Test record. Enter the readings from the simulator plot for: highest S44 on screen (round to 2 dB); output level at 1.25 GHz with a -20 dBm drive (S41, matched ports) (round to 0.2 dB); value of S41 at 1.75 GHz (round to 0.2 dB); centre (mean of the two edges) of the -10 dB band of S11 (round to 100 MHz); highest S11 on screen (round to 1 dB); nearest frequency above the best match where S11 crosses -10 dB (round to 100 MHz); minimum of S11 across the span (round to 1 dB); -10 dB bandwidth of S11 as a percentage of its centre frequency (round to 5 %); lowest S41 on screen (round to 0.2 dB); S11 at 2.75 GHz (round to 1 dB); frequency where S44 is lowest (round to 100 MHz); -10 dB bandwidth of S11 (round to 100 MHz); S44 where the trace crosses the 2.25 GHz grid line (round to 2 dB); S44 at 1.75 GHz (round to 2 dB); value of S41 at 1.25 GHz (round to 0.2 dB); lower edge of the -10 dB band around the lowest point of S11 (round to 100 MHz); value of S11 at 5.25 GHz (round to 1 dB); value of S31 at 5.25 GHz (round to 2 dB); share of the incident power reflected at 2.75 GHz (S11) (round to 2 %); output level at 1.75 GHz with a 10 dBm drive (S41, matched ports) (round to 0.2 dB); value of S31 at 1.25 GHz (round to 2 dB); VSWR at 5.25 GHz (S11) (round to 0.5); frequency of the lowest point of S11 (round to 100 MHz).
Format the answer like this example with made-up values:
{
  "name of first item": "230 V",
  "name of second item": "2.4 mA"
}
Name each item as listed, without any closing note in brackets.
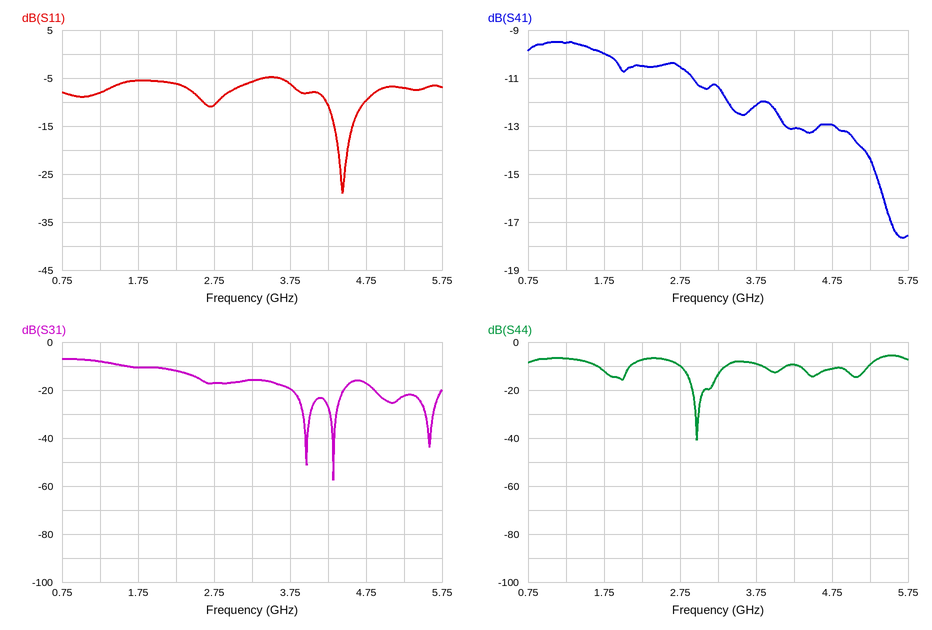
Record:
{
  "highest S44 on screen": "-6 dB",
  "output level at 1.25 GHz with a -20 dBm drive (S41, matched ports)": "-29.6 dBm",
  "value of S41 at 1.75 GHz": "-10.0 dB",
  "centre (mean of the two edges) of the -10 dB band of S11": "4.5 GHz",
  "highest S11 on screen": "-5 dB",
  "nearest frequency above the best match where S11 crosses -10 dB": "4.7 GHz",
  "minimum of S11 across the span": "-29 dB",
  "-10 dB bandwidth of S11 as a percentage of its centre frequency": "10 %",
  "lowest S41 on screen": "-17.6 dB",
  "S11 at 2.75 GHz": "-11 dB",
  "frequency where S44 is lowest": "3.0 GHz",
  "-10 dB bandwidth of S11": "500 MHz",
  "S44 where the trace crosses the 2.25 GHz grid line": "-8 dB",
  "S44 at 1.75 GHz": "-12 dB",
  "value of S41 at 1.25 GHz": "-9.6 dB",
  "lower edge of the -10 dB band around the lowest point of S11": "4.2 GHz",
  "value of S11 at 5.25 GHz": "-7 dB",
  "value of S31 at 5.25 GHz": "-22 dB",
  "share of the incident power reflected at 2.75 GHz (S11)": "8 %",
  "output level at 1.75 GHz with a 10 dBm drive (S41, matched ports)": "0.0 dBm",
  "value of S31 at 1.25 GHz": "-8 dB",
  "VSWR at 5.25 GHz (S11)": "2.5",
  "frequency of the lowest point of S11": "4.4 GHz"
}
